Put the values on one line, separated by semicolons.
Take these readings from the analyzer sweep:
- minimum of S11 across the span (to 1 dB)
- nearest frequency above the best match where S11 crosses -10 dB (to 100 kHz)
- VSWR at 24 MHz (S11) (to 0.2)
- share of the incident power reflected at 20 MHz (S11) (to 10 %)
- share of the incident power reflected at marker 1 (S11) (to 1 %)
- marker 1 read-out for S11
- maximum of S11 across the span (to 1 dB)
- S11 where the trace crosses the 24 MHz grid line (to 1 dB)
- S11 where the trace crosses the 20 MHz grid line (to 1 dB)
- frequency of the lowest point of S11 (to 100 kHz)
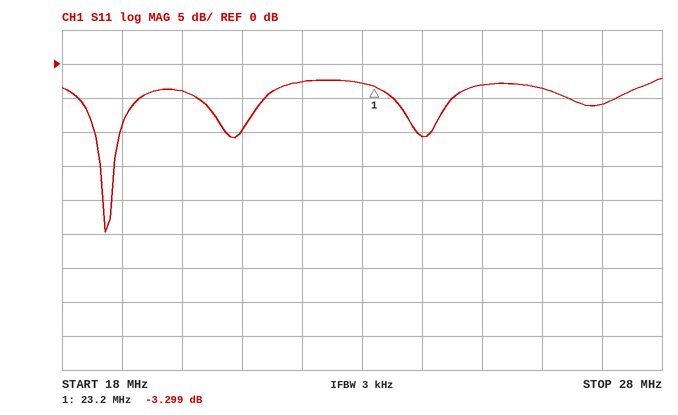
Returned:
-25 dB; 19.0 MHz; 1.8; 40 %; 47 %; -3.299 dB; -2 dB; -11 dB; -4 dB; 18.7 MHz
